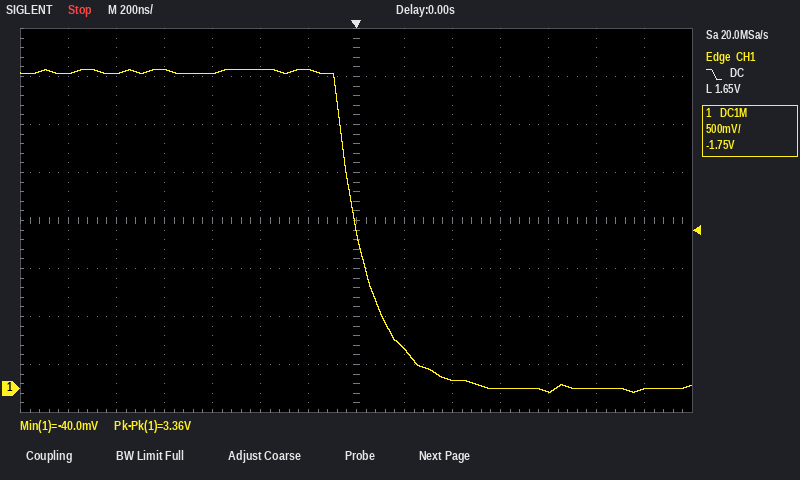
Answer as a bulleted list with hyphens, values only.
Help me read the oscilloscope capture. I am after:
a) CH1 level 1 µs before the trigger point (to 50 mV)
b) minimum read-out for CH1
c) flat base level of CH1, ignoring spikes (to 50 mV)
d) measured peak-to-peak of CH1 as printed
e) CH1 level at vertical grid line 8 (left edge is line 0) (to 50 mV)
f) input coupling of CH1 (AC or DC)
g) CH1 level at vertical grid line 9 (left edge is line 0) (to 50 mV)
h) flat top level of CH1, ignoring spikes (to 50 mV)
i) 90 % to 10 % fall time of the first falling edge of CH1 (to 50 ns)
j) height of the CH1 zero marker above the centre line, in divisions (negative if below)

- 3.30 V
- -40.0 mV
- 0 mV
- 3.36 V
- 400 mV
- DC
- 100 mV
- 3.30 V
- 300 ns
- -3.5 div
